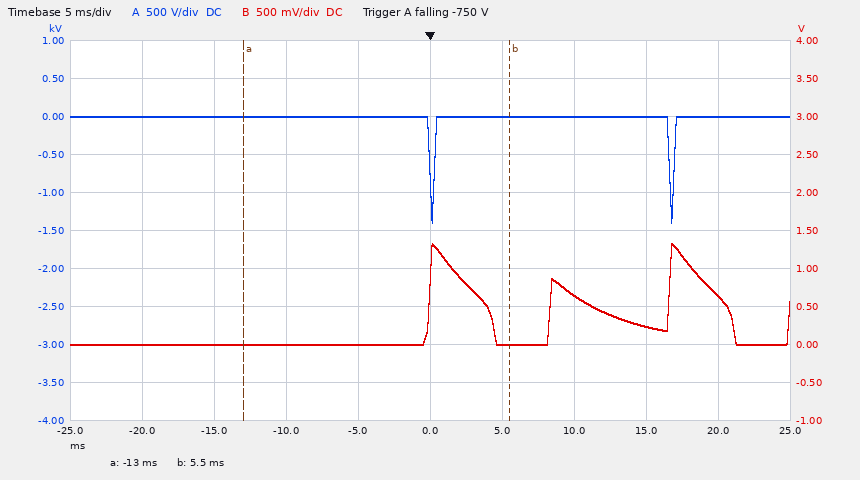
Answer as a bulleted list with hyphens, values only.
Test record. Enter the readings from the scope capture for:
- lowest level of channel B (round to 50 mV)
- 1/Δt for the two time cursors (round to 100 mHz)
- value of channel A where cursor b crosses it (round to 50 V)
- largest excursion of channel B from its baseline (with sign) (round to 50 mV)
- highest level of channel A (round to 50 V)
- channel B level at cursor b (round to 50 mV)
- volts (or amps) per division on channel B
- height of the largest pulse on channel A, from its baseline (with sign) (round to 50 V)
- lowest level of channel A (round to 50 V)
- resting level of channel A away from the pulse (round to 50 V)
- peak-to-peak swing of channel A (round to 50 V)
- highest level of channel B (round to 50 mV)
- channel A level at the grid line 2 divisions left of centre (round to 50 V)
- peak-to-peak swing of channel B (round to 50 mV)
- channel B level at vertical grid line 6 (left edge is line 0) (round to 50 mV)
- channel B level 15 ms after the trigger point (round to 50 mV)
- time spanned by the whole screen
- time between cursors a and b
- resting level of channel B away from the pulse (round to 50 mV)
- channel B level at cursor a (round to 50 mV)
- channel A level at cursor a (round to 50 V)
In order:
- 0 mV
- 54.1 Hz
- 0 V
- +1.35 V
- 0 V
- 0 mV
- 500 mV
- -1.40 kV
- -1.40 kV
- 0 V
- 1.40 kV
- 1.35 V
- 0 V
- 1.35 V
- 0 mV
- 250 mV
- 50 ms
- 18.5 ms
- 0 mV
- 0 mV
- 0 V
